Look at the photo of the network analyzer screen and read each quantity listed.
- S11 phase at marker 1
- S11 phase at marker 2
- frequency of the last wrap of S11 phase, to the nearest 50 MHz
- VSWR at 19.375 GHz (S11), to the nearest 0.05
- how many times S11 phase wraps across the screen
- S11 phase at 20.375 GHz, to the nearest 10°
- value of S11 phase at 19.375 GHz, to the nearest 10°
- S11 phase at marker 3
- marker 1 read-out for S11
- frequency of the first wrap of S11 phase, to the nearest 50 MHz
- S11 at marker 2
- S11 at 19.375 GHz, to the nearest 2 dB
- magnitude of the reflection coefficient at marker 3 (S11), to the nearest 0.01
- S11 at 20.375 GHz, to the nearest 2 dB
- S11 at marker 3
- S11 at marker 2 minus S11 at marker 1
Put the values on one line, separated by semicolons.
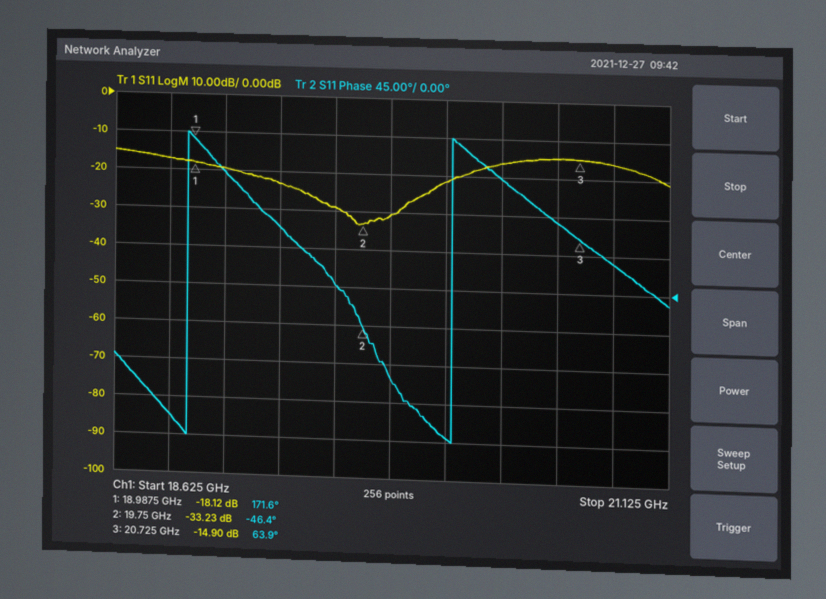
171.6°; -46.4°; 20.15 GHz; 1.15; 2; 130°; 70°; 63.9°; -18.12 dB; 18.95 GHz; -33.23 dB; -24 dB; 0.18; -16 dB; -14.90 dB; -15.11 dB
